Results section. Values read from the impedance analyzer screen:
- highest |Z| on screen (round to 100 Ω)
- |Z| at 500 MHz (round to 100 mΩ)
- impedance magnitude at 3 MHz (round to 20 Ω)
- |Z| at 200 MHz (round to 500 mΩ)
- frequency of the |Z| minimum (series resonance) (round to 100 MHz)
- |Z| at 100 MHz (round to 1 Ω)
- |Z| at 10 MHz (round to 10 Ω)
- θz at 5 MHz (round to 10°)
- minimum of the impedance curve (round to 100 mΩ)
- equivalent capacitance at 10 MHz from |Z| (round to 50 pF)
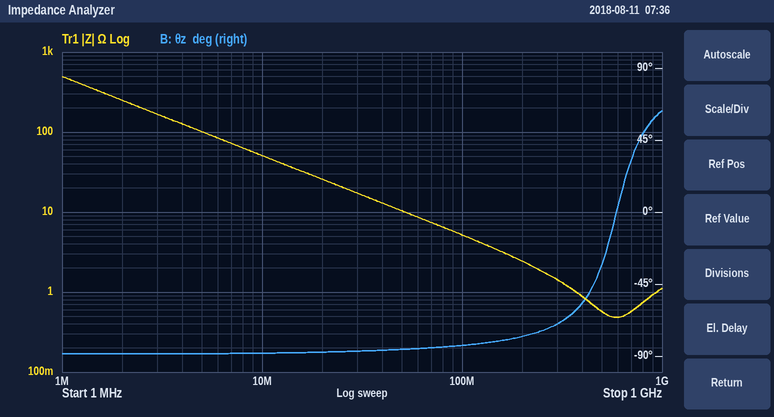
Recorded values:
500 Ω
600 mΩ
160 Ω
2.5 Ω
600 MHz
5 Ω
50 Ω
-90°
500 mΩ
300 pF
